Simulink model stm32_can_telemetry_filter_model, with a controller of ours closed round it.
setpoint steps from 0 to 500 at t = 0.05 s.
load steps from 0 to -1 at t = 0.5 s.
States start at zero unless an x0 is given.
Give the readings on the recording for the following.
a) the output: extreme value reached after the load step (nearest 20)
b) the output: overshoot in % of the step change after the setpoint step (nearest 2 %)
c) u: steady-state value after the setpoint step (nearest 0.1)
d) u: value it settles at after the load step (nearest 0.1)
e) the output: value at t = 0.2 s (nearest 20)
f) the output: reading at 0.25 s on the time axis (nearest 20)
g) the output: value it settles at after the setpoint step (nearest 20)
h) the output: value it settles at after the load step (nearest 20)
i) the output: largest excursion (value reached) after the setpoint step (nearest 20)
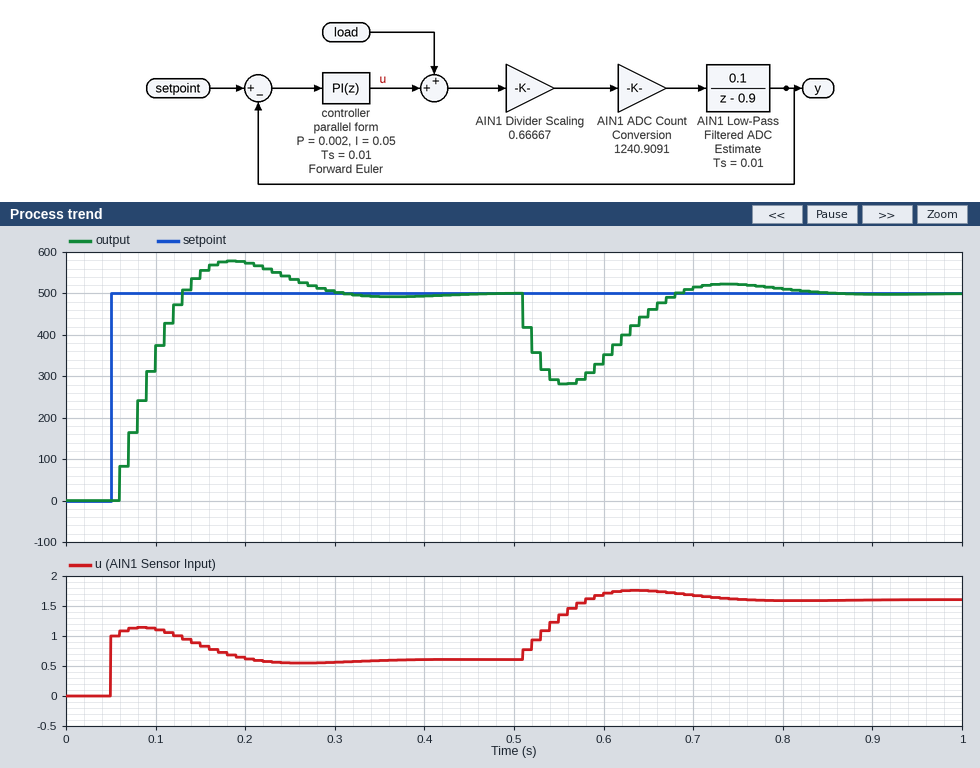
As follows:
280
16 %
0.6
1.6
580
540
500
500
580
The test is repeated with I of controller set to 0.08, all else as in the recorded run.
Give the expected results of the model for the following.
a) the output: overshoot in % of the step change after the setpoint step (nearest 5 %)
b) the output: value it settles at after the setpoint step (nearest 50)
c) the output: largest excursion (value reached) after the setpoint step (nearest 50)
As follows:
30 %
500
650
